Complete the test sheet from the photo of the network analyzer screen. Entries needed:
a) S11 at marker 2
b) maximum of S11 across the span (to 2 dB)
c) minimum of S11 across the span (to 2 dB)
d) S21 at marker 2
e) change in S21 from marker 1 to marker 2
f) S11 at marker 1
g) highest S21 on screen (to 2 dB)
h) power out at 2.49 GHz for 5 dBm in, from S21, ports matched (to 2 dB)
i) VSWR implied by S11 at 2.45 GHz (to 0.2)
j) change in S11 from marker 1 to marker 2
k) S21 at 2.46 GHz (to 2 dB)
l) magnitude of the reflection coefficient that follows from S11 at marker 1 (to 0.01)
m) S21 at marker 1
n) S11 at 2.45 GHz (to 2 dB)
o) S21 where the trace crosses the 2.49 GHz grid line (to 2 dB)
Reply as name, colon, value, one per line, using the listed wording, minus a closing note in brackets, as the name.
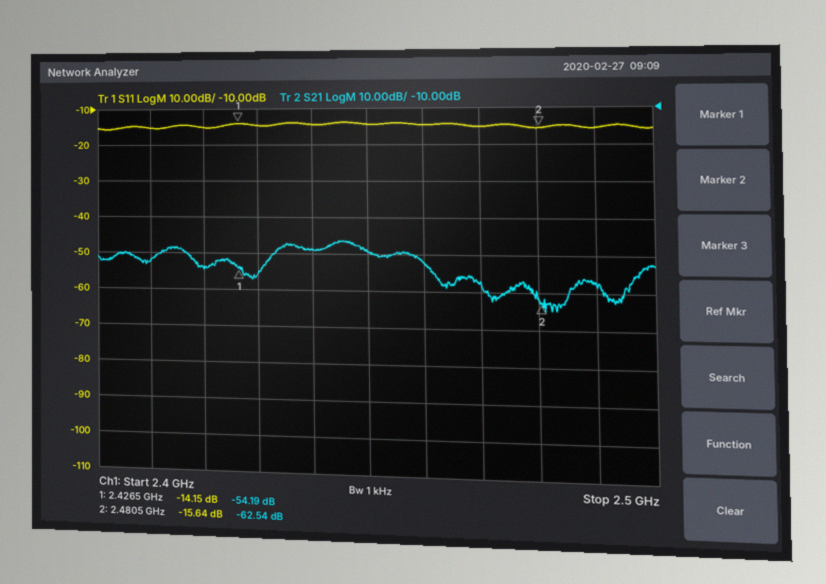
S11 at marker 2: -15.64 dB
maximum of S11 across the span: -14 dB
minimum of S11 across the span: -16 dB
S21 at marker 2: -62.54 dB
change in S21 from marker 1 to marker 2: -8.35 dB
S11 at marker 1: -14.15 dB
highest S21 on screen: -46 dB
power out at 2.49 GHz for 5 dBm in, from S21, ports matched: -52 dBm
VSWR implied by S11 at 2.45 GHz: 1.4
change in S11 from marker 1 to marker 2: -1.49 dB
S21 at 2.46 GHz: -52 dB
magnitude of the reflection coefficient that follows from S11 at marker 1: 0.20
S21 at marker 1: -54.19 dB
S11 at 2.45 GHz: -14 dB
S21 where the trace crosses the 2.49 GHz grid line: -58 dB
